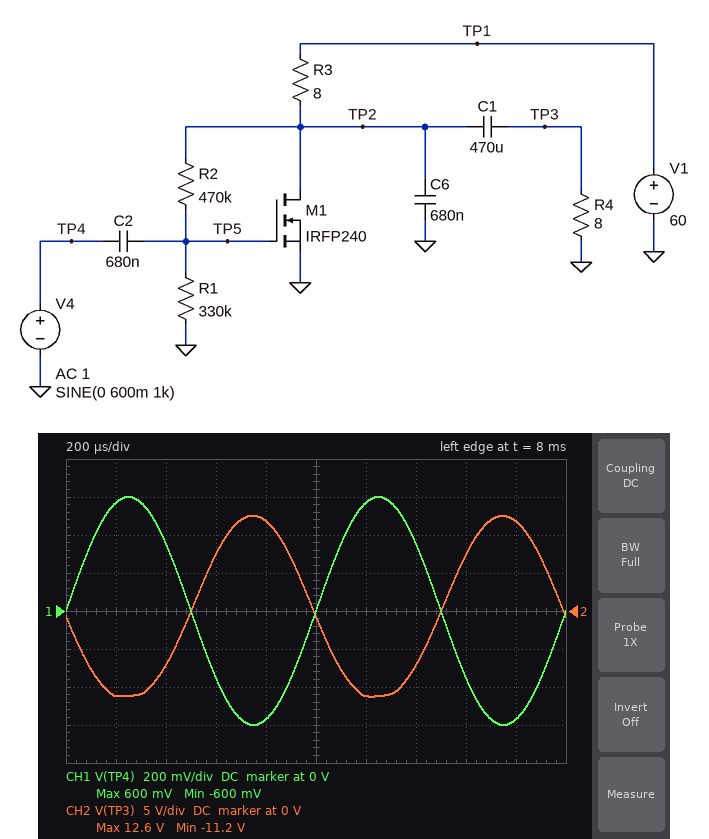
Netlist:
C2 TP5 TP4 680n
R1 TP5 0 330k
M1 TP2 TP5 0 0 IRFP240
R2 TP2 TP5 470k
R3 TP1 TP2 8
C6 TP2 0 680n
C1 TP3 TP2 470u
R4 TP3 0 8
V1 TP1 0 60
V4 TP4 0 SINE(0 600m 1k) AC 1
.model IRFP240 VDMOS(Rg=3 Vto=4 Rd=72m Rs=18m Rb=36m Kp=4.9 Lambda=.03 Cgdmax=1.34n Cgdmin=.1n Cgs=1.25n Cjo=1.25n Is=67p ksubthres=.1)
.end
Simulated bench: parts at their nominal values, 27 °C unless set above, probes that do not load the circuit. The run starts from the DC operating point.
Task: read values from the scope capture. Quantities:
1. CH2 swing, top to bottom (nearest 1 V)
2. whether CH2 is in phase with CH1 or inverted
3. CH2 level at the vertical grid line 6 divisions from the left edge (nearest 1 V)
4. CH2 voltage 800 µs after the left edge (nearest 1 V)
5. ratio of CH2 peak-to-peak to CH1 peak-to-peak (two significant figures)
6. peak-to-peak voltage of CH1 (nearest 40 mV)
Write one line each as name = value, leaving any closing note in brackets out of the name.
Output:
CH2 swing, top to bottom = 24 V
whether CH2 is in phase with CH1 or inverted = inverted
CH2 level at the vertical grid line 6 divisions from the left edge = -11 V
CH2 voltage 800 µs after the left edge = 12 V
ratio of CH2 peak-to-peak to CH1 peak-to-peak = 20
peak-to-peak voltage of CH1 = 1.20 V
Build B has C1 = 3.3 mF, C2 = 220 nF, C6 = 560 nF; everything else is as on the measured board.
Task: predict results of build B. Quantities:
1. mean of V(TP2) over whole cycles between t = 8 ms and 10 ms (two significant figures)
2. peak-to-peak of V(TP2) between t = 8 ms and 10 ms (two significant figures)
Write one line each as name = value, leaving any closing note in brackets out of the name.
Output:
mean of V(TP2) over whole cycles between t = 8 ms and 10 ms = 13 V
peak-to-peak of V(TP2) between t = 8 ms and 10 ms = 23 V
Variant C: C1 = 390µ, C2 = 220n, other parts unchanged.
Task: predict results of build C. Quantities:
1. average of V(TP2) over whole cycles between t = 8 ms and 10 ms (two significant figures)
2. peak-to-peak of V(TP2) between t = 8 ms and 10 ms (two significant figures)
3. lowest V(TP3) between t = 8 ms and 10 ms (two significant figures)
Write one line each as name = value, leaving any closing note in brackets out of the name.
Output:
average of V(TP2) over whole cycles between t = 8 ms and 10 ms = 13 V
peak-to-peak of V(TP2) between t = 8 ms and 10 ms = 23 V
lowest V(TP3) between t = 8 ms and 10 ms = -11 V
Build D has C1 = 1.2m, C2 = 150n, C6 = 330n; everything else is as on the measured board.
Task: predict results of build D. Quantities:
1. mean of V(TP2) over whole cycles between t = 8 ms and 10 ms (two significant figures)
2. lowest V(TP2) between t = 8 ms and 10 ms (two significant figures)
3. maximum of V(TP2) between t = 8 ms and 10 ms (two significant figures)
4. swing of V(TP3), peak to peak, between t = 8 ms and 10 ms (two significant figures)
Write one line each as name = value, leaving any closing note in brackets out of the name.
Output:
mean of V(TP2) over whole cycles between t = 8 ms and 10 ms = 13 V
lowest V(TP2) between t = 8 ms and 10 ms = 2.4 V
maximum of V(TP2) between t = 8 ms and 10 ms = 25 V
swing of V(TP3), peak to peak, between t = 8 ms and 10 ms = 23 V
